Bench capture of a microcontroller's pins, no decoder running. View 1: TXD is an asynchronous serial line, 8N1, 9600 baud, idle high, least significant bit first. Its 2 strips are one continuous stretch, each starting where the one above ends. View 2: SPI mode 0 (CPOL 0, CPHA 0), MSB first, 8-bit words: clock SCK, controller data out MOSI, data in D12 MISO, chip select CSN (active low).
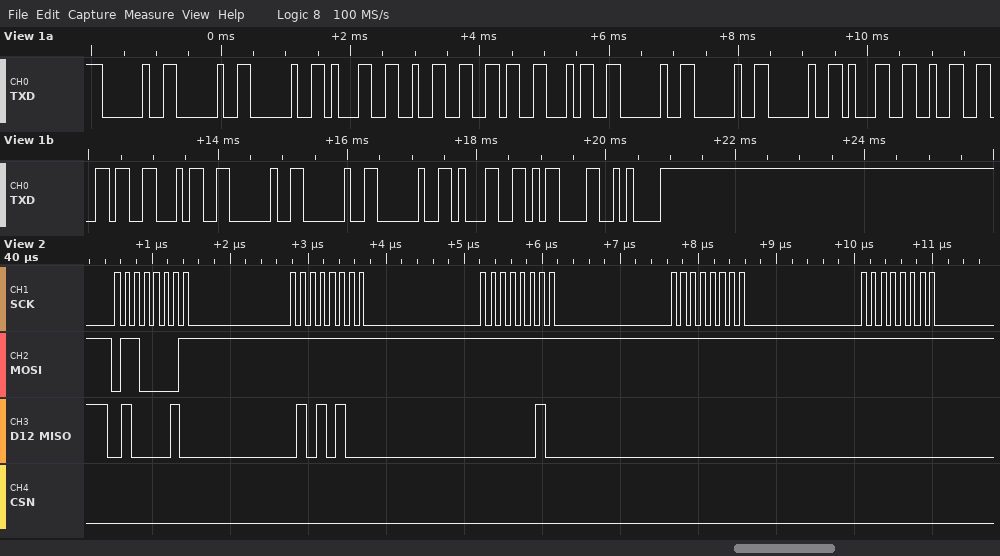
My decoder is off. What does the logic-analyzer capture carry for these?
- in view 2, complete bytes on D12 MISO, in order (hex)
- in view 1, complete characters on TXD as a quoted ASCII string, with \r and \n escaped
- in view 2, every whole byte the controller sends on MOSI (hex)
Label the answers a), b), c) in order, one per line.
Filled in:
a) 42 54 02 00 00
b) "   1264   1264   1\r\n"
c) 61 FF FF FF FF
